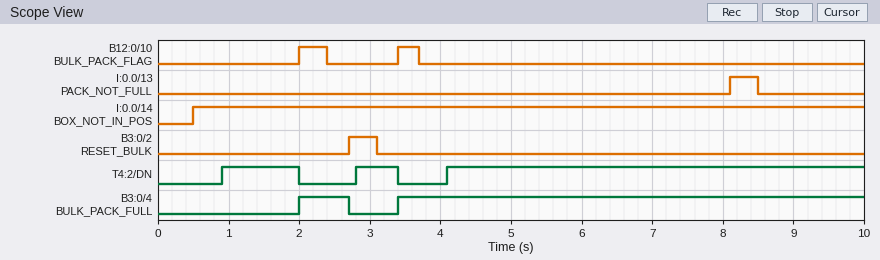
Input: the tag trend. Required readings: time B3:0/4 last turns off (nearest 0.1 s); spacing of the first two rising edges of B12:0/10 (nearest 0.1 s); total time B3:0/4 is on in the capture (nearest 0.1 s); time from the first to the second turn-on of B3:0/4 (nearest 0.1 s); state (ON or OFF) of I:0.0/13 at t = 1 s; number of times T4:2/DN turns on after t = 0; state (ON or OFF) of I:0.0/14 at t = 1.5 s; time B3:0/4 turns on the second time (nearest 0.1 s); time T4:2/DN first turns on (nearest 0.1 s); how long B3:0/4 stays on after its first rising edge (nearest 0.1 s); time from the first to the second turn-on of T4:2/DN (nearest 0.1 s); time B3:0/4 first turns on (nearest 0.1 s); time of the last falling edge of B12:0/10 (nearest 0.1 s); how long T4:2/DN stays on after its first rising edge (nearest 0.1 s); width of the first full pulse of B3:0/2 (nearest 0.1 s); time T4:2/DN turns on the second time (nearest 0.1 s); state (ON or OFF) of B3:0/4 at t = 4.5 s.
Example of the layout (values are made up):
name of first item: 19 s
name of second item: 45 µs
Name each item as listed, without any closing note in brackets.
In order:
time B3:0/4 last turns off: 2.7 s
spacing of the first two rising edges of B12:0/10: 1.4 s
total time B3:0/4 is on in the capture: 7.3 s
time from the first to the second turn-on of B3:0/4: 1.4 s
state (ON or OFF) of I:0.0/13 at t = 1 s: OFF
number of times T4:2/DN turns on after t = 0: 3
state (ON or OFF) of I:0.0/14 at t = 1.5 s: ON
time B3:0/4 turns on the second time: 3.4 s
time T4:2/DN first turns on: 0.9 s
how long B3:0/4 stays on after its first rising edge: 0.7 s
time from the first to the second turn-on of T4:2/DN: 1.9 s
time B3:0/4 first turns on: 2.0 s
time of the last falling edge of B12:0/10: 3.7 s
how long T4:2/DN stays on after its first rising edge: 1.1 s
width of the first full pulse of B3:0/2: 0.4 s
time T4:2/DN turns on the second time: 2.8 s
state (ON or OFF) of B3:0/4 at t = 4.5 s: ON
